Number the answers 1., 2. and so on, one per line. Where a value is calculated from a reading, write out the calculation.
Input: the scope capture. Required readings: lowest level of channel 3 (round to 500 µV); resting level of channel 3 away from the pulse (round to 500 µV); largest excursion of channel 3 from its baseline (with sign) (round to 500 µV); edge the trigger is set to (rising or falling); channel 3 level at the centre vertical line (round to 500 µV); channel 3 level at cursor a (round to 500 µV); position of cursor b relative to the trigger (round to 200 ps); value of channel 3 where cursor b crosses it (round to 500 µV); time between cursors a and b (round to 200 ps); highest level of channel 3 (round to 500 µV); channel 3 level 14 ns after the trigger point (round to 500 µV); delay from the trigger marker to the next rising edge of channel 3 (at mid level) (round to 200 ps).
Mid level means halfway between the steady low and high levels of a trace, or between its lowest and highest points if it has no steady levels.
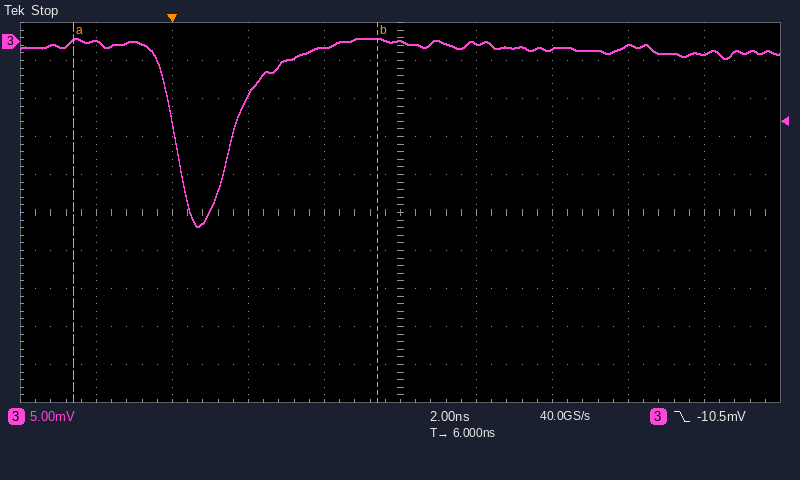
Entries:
1. -24.5 mV
2. -1.0 mV
3. -24.5 mV − (-1.0 mV) = -23.5 mV
4. falling
5. 0.0 mV
6. 0.0 mV
7. +5.4 ns
8. 500 µV
9. 8.0 ns
10. 500 µV
11. -1.5 mV
12. 1.6 ns
